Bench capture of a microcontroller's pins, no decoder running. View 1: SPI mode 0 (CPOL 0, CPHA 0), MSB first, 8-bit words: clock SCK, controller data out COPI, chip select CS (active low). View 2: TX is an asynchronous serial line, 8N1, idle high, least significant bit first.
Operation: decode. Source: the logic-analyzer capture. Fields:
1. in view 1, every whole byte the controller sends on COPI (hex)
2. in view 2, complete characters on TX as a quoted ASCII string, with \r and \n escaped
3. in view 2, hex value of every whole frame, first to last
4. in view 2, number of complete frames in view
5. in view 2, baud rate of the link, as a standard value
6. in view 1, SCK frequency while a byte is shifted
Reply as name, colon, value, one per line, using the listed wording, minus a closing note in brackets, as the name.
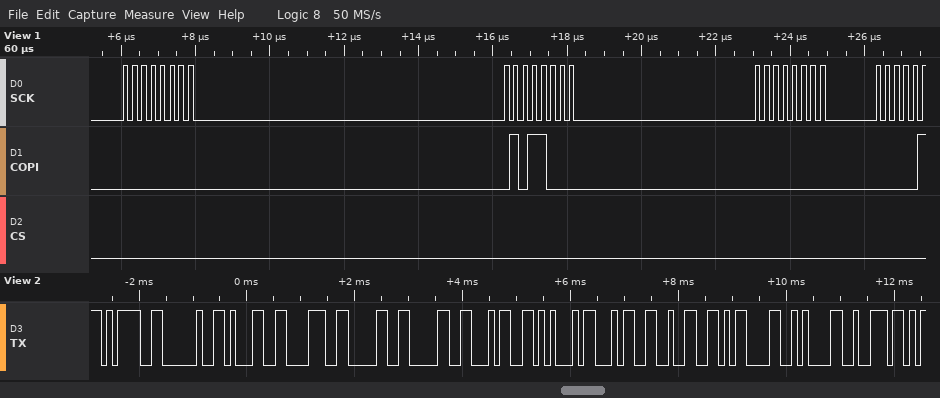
in view 1, every whole byte the controller sends on COPI: 00 58 00
in view 2, complete characters on TX as a quoted ASCII string, with \r and \n escaped: "= 18004E42\r\nr"
in view 2, hex value of every whole frame, first to last: 0x3D 0x20 0x31 0x38 0x30 0x30 0x34 0x45 0x34 0x32 0x0D 0x0A 0x72
in view 2, number of complete frames in view: 13
in view 2, baud rate of the link, as a standard value: 9600 baud
in view 1, SCK frequency while a byte is shifted: 4 MHz
